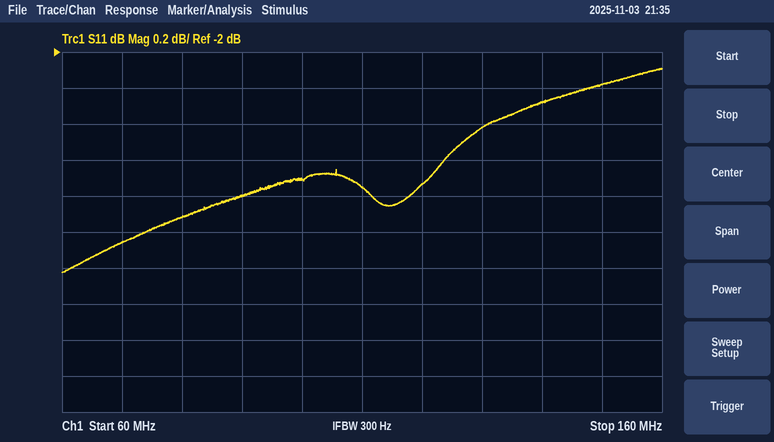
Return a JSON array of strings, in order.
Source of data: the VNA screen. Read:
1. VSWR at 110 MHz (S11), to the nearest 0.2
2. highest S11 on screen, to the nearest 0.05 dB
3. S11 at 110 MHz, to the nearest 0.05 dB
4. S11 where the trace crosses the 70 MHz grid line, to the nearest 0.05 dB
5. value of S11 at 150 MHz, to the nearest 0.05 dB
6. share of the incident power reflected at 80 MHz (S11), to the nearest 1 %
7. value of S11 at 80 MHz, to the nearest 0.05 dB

["6.4", "-2.10 dB", "-2.75 dB", "-3.05 dB", "-2.20 dB", "51 %", "-2.90 dB"]
